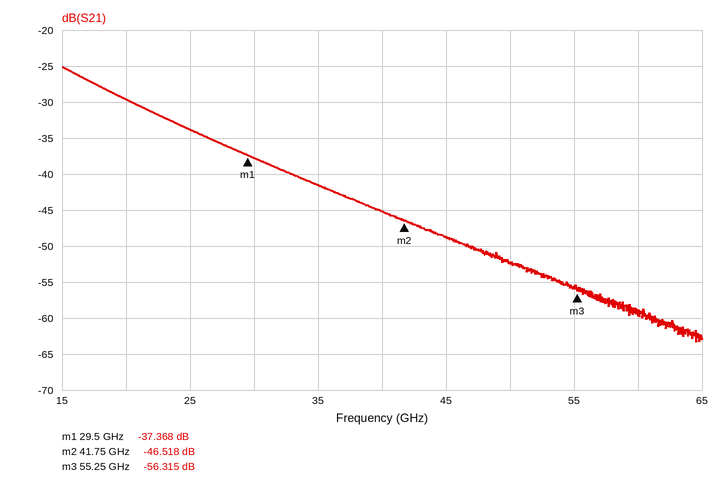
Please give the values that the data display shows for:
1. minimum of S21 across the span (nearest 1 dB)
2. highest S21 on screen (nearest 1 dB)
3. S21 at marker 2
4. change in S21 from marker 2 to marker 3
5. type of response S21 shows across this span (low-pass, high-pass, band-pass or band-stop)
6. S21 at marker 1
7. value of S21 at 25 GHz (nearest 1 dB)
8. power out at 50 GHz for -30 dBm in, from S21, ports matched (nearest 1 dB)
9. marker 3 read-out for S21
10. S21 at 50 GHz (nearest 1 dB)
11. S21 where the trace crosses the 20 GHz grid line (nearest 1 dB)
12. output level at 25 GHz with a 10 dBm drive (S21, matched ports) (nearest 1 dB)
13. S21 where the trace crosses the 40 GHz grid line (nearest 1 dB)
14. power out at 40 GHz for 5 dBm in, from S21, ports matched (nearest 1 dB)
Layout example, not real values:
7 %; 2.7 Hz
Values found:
-63 dB; -25 dB; -46.518 dB; -9.797 dB; low-pass; -37.368 dB; -34 dB; -82 dBm; -56.315 dB; -52 dB; -30 dB; -24 dBm; -45 dB; -40 dBm
